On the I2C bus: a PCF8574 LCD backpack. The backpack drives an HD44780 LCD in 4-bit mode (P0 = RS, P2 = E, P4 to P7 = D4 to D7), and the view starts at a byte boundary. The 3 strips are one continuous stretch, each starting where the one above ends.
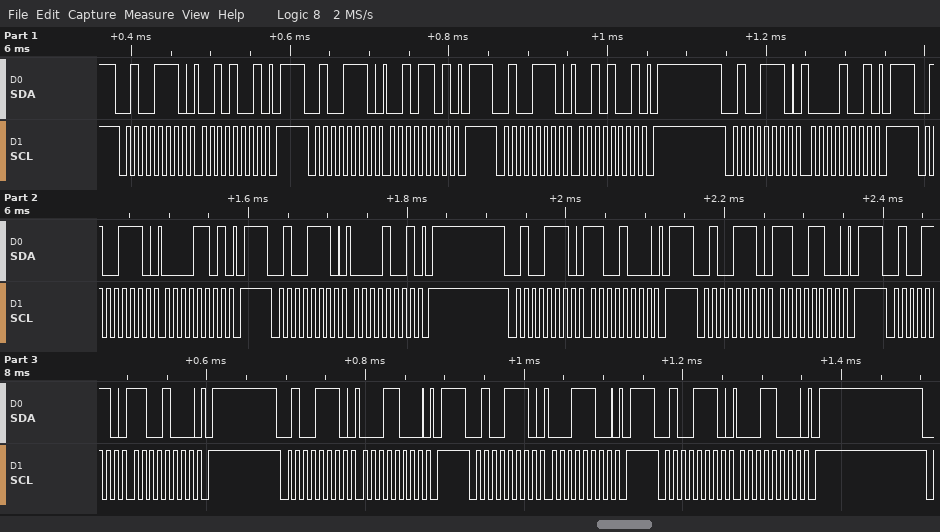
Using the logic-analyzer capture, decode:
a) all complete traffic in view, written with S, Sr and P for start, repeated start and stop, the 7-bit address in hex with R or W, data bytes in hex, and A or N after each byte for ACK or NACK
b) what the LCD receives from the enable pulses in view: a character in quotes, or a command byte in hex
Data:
S 27W A 29 A P S 27W A 2D A P S 27W A 29 A P S 27W A 09 A P S 27W A 0D A P S 27W A 09 A P S 27W A C8 A P S 27W A CC A P S 27W A C8 A P S 27W A 18 A P S 27W A 1C A P S 27W A 18 A P
' ' 0xC1
